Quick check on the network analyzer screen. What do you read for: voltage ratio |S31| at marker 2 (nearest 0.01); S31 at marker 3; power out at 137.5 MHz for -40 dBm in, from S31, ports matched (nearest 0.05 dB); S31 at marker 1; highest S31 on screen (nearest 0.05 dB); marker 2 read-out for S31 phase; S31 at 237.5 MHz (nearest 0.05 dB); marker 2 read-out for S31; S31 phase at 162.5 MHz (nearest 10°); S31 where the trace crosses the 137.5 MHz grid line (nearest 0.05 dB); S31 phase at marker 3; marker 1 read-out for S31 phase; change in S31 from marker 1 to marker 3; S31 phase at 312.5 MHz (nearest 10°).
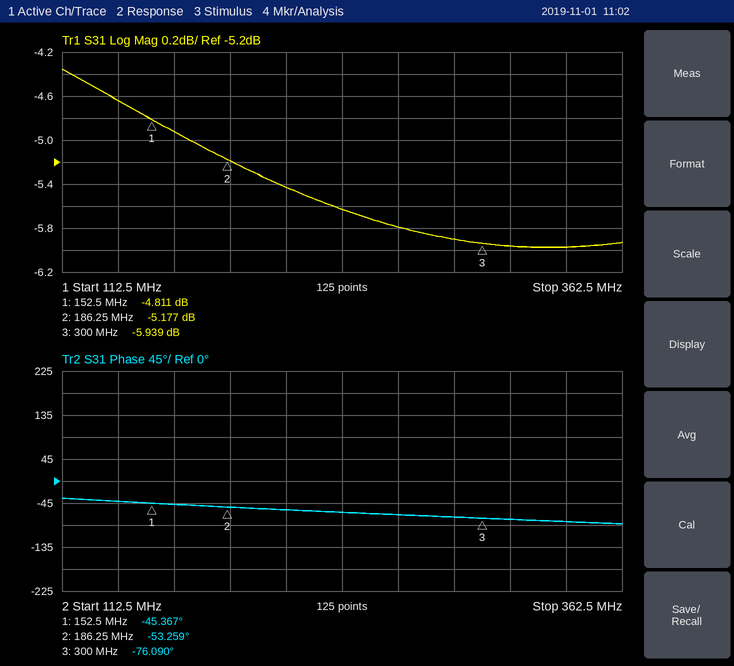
0.55
-5.939 dB
-44.65 dBm
-4.811 dB
-4.35 dB
-53.259°
-5.65 dB
-5.177 dB
-50°
-4.65 dB
-76.090°
-45.367°
-1.128 dB
-80°
